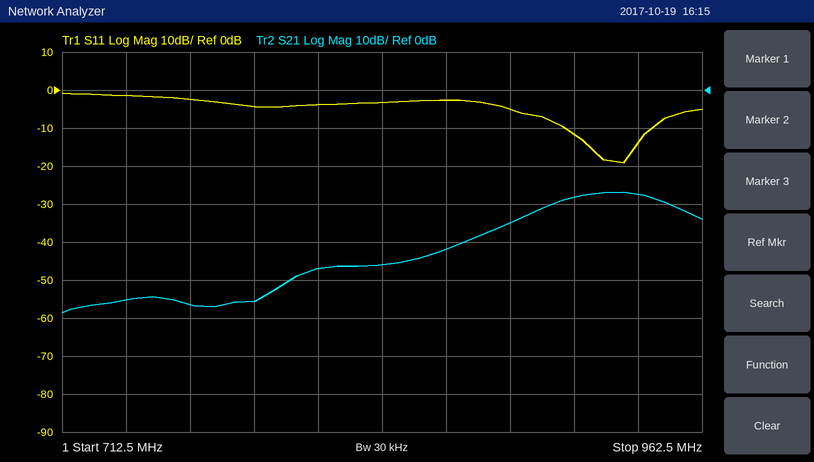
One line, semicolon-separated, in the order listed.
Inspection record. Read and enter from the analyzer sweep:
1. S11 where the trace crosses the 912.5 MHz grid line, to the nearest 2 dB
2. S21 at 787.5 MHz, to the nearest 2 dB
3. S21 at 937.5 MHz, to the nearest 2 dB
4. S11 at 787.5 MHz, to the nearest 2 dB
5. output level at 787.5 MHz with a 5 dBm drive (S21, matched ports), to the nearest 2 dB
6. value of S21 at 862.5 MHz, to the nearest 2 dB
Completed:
-12 dB; -56 dB; -28 dB; -4 dB; -50 dBm; -42 dB
